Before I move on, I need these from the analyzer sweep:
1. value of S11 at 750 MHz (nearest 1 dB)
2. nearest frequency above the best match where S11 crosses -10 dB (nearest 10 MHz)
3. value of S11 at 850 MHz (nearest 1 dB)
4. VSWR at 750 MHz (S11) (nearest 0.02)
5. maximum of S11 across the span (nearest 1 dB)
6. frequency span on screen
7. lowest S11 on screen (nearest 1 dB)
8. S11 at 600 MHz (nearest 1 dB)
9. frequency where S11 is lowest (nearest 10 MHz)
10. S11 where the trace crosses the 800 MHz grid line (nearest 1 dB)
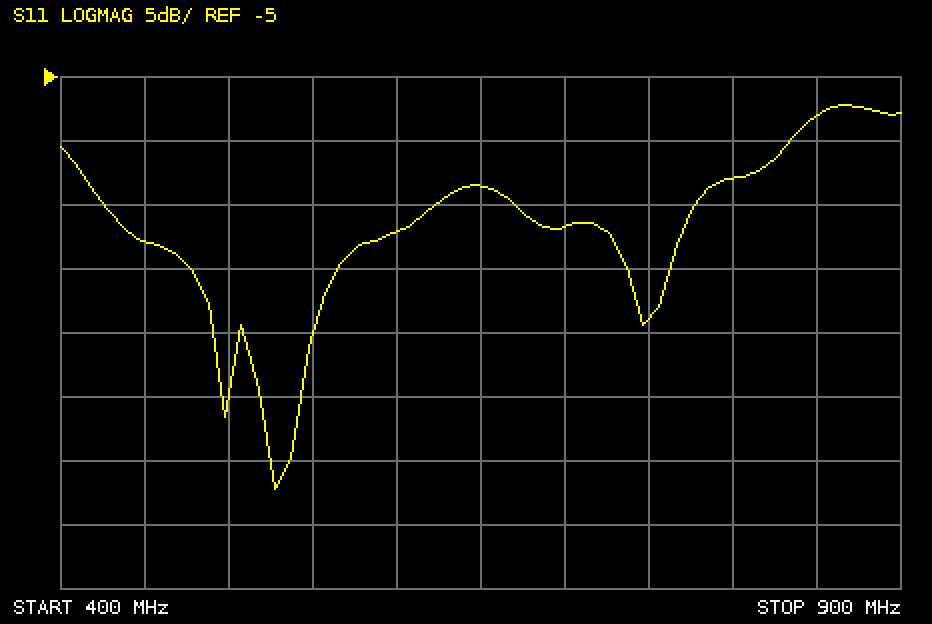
-24 dB
830 MHz
-8 dB
1.14
-7 dB
500 MHz
-37 dB
-17 dB
530 MHz
-13 dB
